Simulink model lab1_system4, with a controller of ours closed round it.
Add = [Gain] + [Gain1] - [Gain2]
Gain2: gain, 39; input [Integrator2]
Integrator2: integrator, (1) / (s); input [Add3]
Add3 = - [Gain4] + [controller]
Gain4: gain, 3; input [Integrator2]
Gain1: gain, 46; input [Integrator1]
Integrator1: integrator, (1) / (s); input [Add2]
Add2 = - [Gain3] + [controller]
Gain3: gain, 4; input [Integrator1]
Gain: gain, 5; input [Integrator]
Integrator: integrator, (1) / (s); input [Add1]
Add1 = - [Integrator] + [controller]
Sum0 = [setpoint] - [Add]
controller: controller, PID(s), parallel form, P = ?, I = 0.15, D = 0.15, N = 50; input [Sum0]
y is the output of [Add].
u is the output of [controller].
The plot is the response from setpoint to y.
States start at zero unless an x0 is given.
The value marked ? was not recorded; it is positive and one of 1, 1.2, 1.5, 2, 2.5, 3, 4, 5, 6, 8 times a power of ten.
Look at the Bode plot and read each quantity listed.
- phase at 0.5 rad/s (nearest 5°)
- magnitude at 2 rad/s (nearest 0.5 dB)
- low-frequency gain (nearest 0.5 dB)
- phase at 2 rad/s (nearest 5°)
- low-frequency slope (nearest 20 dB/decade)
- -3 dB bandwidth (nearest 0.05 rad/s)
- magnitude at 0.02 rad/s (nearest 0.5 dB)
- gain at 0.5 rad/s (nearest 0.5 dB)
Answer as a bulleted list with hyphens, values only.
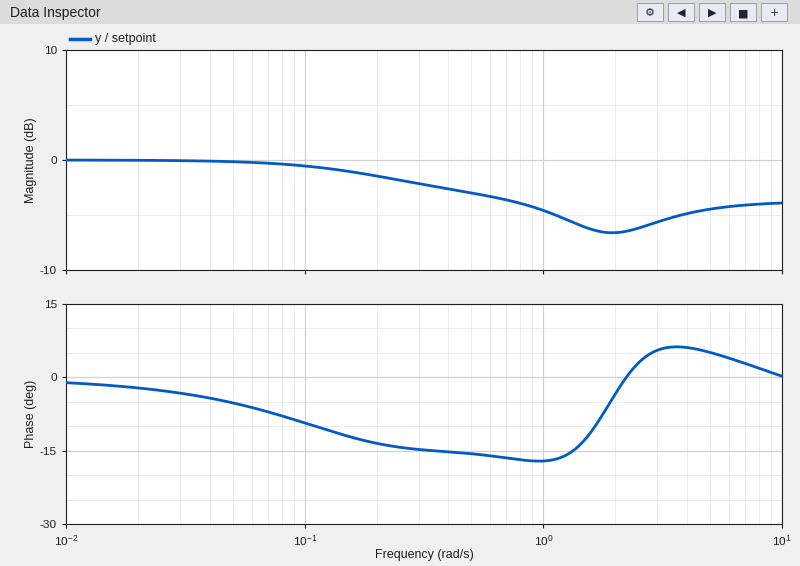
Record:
- -15°
- -6.5 dB
- 0.0 dB
- -5°
- 0 dB/decade
- 0.50 rad/s
- 0.0 dB
- -3.0 dB
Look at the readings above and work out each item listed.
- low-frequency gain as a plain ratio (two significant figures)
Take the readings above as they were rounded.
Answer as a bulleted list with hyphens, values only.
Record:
- 1.0
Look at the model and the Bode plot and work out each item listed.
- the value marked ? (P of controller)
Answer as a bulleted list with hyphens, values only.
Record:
- 0.6
